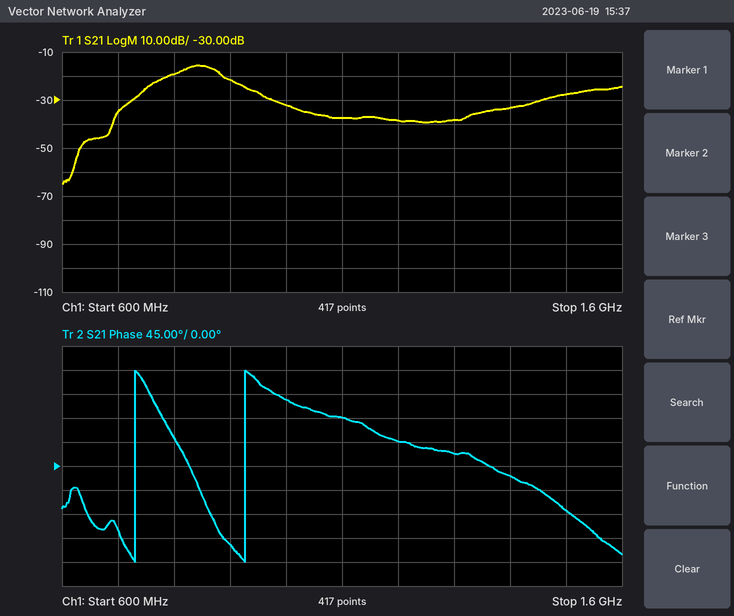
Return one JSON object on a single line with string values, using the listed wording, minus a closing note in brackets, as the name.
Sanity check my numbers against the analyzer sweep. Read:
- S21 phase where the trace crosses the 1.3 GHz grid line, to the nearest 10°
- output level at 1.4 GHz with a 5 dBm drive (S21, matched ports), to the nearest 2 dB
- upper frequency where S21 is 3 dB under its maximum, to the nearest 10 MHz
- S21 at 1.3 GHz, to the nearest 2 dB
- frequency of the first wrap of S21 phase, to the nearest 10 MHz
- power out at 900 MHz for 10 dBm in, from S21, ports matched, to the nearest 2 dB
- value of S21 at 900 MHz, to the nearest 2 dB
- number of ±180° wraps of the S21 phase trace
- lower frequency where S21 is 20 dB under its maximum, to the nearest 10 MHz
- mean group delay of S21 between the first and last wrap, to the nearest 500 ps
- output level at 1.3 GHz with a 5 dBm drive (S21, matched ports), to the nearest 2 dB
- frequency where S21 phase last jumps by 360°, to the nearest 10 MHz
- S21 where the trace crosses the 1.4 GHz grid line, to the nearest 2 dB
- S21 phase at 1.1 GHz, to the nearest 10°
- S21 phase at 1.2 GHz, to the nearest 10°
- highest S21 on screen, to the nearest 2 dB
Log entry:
{"S21 phase where the trace crosses the 1.3 GHz grid line, to the nearest 10°": "20°", "output level at 1.4 GHz with a 5 dBm drive (S21, matched ports), to the nearest 2 dB": "-28 dBm", "upper frequency where S21 is 3 dB under its maximum, to the nearest 10 MHz": "880 MHz", "S21 at 1.3 GHz, to the nearest 2 dB": "-38 dB", "frequency of the first wrap of S21 phase, to the nearest 10 MHz": "730 MHz", "power out at 900 MHz for 10 dBm in, from S21, ports matched, to the nearest 2 dB": "-12 dBm", "value of S21 at 900 MHz, to the nearest 2 dB": "-22 dB", "number of ±180° wraps of the S21 phase trace": "2", "lower frequency where S21 is 20 dB under its maximum, to the nearest 10 MHz": "700 MHz", "mean group delay of S21 between the first and last wrap, to the nearest 500 ps": "5.0 ns", "output level at 1.3 GHz with a 5 dBm drive (S21, matched ports), to the nearest 2 dB": "-34 dBm", "frequency where S21 phase last jumps by 360°, to the nearest 10 MHz": "930 MHz", "S21 where the trace crosses the 1.4 GHz grid line, to the nearest 2 dB": "-34 dB", "S21 phase at 1.1 GHz, to the nearest 10°": "90°", "S21 phase at 1.2 GHz, to the nearest 10°": "50°", "highest S21 on screen, to the nearest 2 dB": "-16 dB"}
